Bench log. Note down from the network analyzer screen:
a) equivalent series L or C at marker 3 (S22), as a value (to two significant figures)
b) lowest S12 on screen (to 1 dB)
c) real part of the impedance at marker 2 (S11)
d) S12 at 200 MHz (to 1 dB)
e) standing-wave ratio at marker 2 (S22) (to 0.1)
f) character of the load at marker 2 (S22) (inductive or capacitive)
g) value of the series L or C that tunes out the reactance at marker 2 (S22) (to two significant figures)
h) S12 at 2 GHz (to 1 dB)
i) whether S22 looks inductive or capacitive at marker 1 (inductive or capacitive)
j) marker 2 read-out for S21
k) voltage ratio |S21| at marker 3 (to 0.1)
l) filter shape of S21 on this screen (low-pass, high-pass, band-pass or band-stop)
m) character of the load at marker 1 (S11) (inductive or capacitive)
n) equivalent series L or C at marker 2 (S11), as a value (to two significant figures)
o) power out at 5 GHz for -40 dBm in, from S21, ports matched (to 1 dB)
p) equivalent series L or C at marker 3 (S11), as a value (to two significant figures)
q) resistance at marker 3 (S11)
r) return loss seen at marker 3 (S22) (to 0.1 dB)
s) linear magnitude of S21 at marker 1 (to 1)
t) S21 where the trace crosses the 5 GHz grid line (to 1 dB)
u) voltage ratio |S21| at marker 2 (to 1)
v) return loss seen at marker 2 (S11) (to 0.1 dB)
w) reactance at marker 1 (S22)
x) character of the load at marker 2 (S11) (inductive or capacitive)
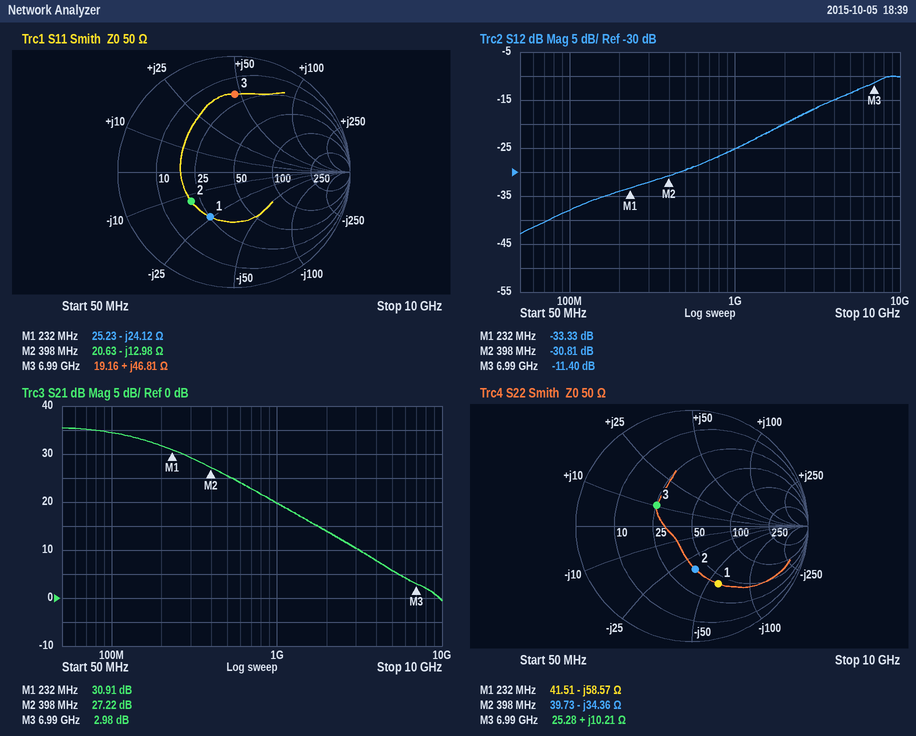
230 pH
-43 dB
20.63 Ω
-34 dB
2.2
capacitive
14 nH
-20 dB
capacitive
27.22 dB
1.4
low-pass
capacitive
31 pF
-34 dBm
1.1 nH
19.16 Ω
9.1 dB
35
6 dB
23
7.0 dB
-58.57 Ω
capacitive
